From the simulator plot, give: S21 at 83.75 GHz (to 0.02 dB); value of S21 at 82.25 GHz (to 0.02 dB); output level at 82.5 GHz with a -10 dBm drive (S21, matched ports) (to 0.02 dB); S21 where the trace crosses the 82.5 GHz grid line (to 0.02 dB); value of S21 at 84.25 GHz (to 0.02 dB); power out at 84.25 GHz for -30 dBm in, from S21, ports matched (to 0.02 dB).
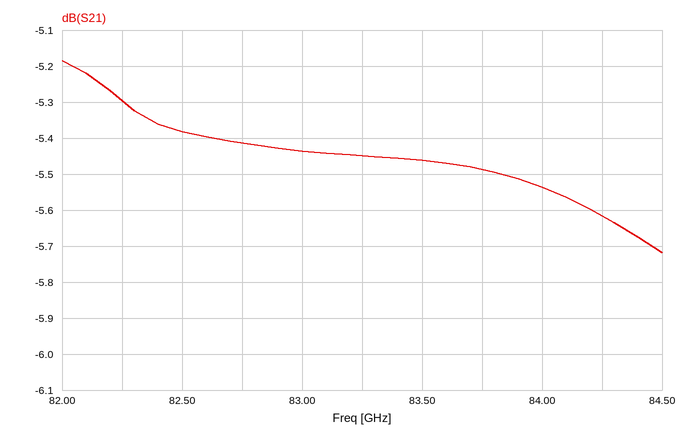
-5.48 dB
-5.30 dB
-15.38 dBm
-5.38 dB
-5.62 dB
-35.62 dBm
